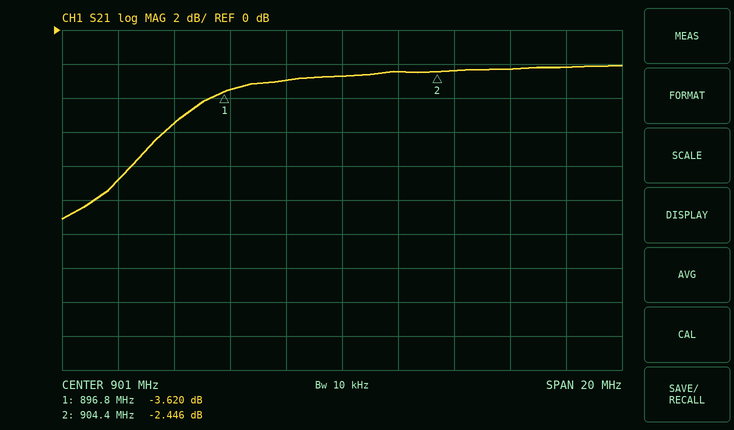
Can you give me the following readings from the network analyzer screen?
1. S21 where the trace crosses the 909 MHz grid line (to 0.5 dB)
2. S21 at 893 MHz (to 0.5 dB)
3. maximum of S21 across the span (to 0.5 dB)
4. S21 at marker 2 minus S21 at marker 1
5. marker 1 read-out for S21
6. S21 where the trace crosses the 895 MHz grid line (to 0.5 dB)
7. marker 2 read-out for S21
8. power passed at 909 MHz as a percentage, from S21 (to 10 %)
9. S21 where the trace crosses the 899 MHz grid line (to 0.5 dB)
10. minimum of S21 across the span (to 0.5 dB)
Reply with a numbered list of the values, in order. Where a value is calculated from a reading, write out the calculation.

1. -2.0 dB
2. -9.0 dB
3. -2.0 dB
4. -2.446 − (-3.62) = 1.174 dB
5. -3.620 dB
6. -5.5 dB
7. -2.446 dB
8. 10^(-2/10) ≈ 63.1 %, so 60 % to the nearest 10 %
9. -3.0 dB
10. -11.0 dB
